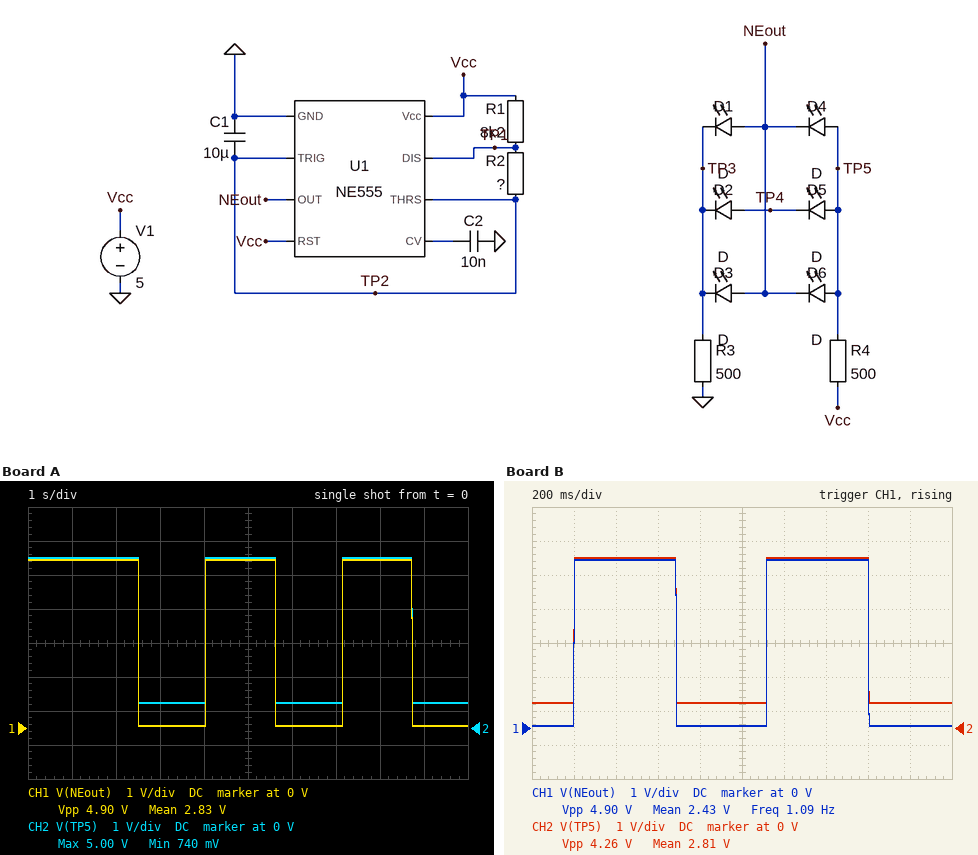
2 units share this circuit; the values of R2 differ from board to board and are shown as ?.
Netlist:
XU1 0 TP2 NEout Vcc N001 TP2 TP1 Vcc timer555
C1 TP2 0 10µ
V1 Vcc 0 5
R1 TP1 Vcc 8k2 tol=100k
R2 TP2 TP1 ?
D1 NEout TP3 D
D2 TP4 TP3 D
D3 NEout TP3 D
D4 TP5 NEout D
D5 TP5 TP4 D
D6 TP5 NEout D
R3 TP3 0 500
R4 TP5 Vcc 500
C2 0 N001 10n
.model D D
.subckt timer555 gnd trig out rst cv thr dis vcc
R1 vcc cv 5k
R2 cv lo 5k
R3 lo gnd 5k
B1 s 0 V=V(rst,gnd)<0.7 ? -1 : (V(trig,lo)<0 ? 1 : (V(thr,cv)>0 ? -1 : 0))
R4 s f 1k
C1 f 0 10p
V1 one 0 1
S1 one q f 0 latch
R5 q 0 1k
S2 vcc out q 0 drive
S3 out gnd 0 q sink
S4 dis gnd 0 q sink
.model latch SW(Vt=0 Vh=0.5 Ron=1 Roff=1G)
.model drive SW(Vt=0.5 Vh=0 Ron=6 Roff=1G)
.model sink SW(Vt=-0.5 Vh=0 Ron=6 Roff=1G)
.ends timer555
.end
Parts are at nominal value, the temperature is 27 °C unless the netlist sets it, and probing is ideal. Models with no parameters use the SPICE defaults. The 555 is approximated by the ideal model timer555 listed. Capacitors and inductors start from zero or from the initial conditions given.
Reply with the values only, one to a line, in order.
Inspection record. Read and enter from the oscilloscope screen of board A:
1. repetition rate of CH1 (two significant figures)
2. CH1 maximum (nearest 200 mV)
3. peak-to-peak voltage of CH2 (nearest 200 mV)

320 mHz
5.0 V
4.2 V
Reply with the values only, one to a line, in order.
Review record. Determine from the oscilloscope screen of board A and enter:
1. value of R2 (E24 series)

220 kΩ
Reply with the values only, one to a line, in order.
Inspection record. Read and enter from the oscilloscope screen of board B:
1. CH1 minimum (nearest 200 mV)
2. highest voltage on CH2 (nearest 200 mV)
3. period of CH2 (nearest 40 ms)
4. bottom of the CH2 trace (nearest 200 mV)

0 V
5.0 V
920 ms
800 mV
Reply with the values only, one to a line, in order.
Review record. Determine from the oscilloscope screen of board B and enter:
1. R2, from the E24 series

62 kΩ
